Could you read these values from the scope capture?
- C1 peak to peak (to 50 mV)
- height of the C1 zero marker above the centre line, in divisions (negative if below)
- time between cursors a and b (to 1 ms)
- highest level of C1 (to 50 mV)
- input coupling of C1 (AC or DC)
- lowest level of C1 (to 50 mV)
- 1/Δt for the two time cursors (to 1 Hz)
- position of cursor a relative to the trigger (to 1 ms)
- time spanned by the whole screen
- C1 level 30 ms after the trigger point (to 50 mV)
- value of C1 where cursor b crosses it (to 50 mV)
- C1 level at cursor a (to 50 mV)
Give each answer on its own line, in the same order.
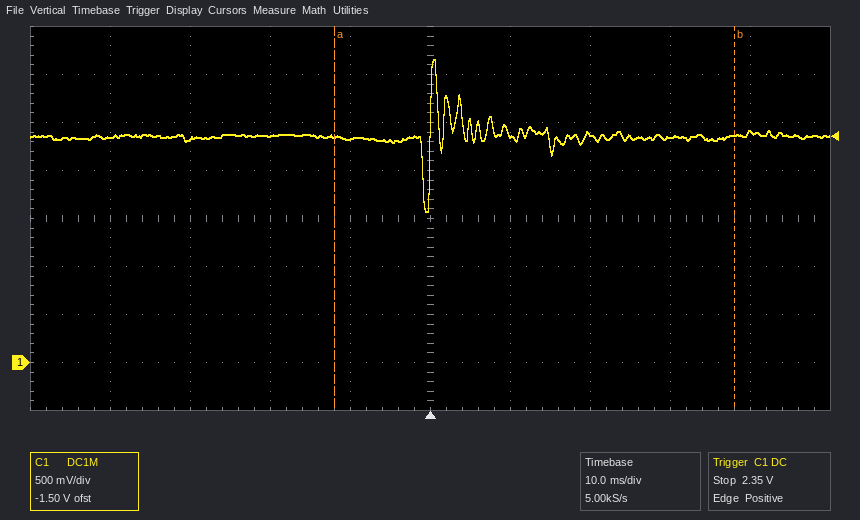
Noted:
1.60 V
-3.0 div
50 ms
3.15 V
DC
1.55 V
20 Hz
-12 ms
100 ms
2.35 V
2.35 V
2.35 V
